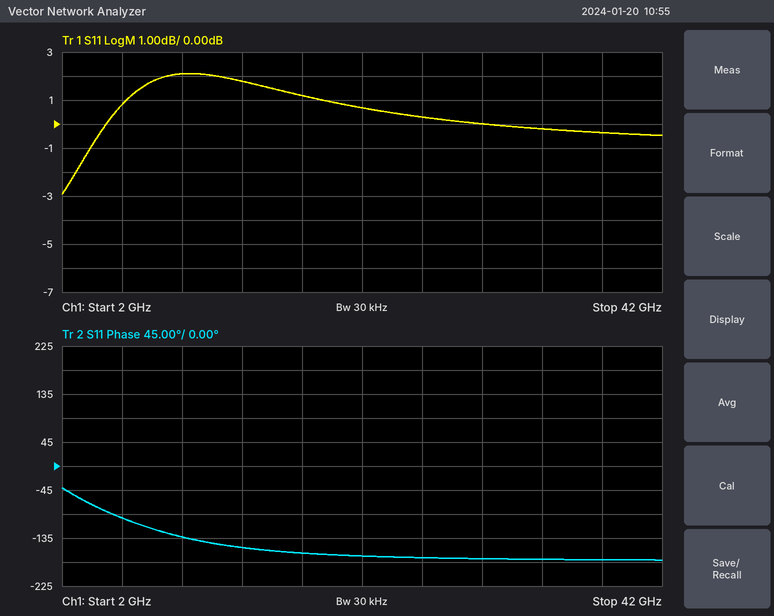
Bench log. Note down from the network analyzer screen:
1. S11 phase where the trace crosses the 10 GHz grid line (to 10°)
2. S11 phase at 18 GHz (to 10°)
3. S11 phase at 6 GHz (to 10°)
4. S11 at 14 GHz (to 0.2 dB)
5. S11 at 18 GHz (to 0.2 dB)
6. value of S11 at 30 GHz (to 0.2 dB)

-130°
-160°
-100°
1.8 dB
1.2 dB
0.0 dB
